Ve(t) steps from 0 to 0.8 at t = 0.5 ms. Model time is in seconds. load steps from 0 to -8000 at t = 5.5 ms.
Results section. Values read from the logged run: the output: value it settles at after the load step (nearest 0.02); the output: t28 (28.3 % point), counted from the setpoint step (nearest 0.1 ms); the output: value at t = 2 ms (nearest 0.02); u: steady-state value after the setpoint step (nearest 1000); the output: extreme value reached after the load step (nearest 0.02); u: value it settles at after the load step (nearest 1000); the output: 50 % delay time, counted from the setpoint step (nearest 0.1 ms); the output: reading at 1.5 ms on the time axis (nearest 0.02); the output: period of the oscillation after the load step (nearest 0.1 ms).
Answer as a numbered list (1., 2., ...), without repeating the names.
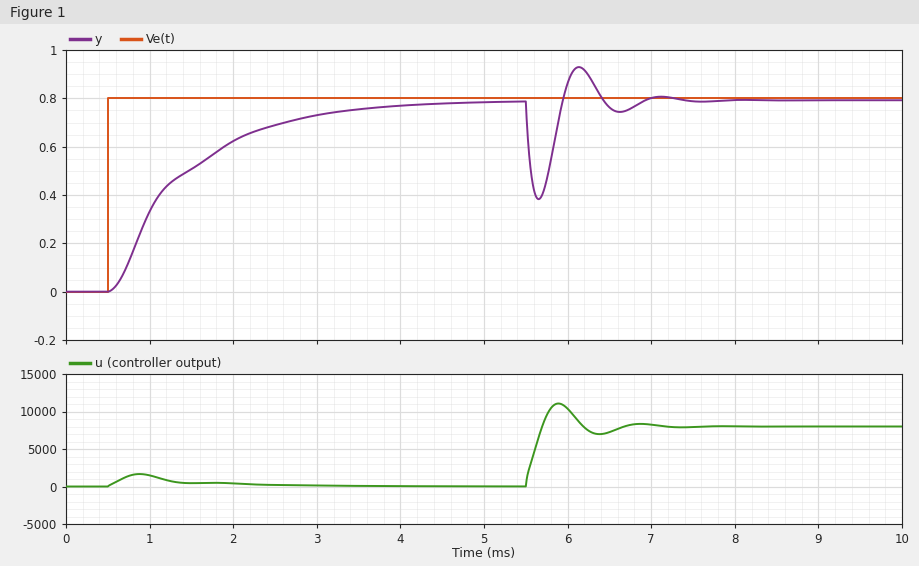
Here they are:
1. 0.80
2. 0.4 ms
3. 0.62
4. 0
5. 0.38
6. 8000
7. 0.6 ms
8. 0.50
9. 1.0 ms
